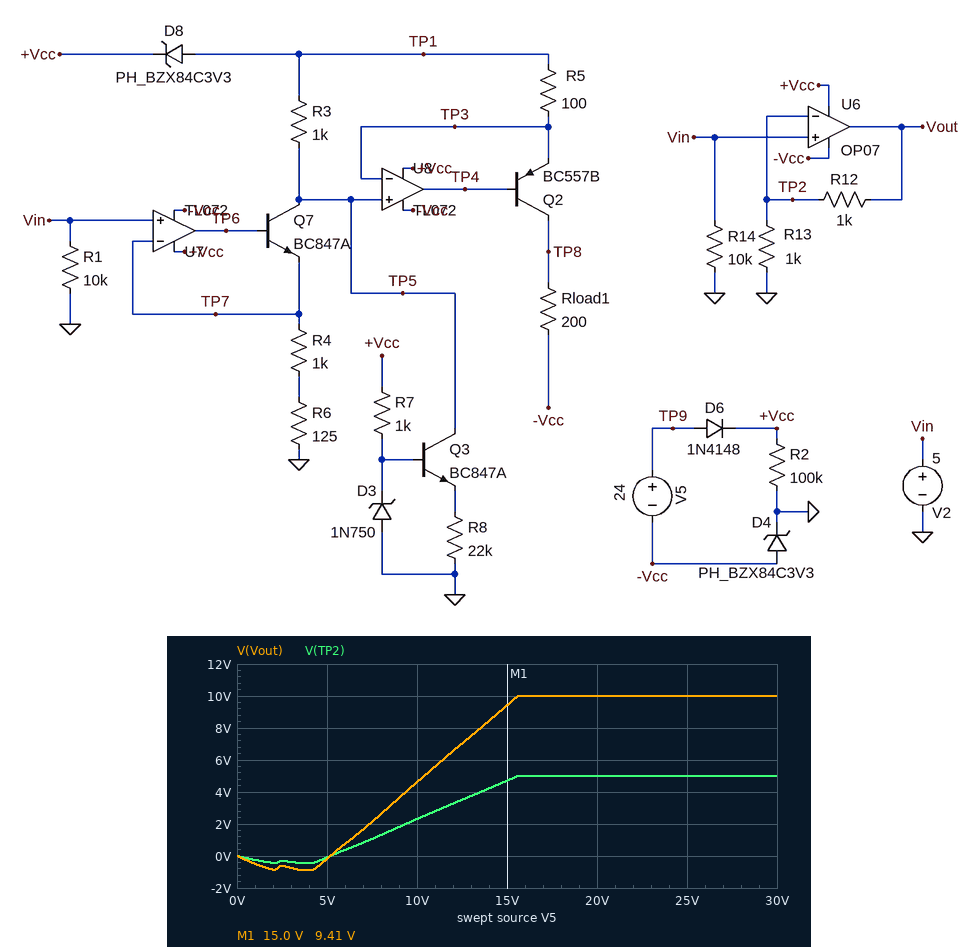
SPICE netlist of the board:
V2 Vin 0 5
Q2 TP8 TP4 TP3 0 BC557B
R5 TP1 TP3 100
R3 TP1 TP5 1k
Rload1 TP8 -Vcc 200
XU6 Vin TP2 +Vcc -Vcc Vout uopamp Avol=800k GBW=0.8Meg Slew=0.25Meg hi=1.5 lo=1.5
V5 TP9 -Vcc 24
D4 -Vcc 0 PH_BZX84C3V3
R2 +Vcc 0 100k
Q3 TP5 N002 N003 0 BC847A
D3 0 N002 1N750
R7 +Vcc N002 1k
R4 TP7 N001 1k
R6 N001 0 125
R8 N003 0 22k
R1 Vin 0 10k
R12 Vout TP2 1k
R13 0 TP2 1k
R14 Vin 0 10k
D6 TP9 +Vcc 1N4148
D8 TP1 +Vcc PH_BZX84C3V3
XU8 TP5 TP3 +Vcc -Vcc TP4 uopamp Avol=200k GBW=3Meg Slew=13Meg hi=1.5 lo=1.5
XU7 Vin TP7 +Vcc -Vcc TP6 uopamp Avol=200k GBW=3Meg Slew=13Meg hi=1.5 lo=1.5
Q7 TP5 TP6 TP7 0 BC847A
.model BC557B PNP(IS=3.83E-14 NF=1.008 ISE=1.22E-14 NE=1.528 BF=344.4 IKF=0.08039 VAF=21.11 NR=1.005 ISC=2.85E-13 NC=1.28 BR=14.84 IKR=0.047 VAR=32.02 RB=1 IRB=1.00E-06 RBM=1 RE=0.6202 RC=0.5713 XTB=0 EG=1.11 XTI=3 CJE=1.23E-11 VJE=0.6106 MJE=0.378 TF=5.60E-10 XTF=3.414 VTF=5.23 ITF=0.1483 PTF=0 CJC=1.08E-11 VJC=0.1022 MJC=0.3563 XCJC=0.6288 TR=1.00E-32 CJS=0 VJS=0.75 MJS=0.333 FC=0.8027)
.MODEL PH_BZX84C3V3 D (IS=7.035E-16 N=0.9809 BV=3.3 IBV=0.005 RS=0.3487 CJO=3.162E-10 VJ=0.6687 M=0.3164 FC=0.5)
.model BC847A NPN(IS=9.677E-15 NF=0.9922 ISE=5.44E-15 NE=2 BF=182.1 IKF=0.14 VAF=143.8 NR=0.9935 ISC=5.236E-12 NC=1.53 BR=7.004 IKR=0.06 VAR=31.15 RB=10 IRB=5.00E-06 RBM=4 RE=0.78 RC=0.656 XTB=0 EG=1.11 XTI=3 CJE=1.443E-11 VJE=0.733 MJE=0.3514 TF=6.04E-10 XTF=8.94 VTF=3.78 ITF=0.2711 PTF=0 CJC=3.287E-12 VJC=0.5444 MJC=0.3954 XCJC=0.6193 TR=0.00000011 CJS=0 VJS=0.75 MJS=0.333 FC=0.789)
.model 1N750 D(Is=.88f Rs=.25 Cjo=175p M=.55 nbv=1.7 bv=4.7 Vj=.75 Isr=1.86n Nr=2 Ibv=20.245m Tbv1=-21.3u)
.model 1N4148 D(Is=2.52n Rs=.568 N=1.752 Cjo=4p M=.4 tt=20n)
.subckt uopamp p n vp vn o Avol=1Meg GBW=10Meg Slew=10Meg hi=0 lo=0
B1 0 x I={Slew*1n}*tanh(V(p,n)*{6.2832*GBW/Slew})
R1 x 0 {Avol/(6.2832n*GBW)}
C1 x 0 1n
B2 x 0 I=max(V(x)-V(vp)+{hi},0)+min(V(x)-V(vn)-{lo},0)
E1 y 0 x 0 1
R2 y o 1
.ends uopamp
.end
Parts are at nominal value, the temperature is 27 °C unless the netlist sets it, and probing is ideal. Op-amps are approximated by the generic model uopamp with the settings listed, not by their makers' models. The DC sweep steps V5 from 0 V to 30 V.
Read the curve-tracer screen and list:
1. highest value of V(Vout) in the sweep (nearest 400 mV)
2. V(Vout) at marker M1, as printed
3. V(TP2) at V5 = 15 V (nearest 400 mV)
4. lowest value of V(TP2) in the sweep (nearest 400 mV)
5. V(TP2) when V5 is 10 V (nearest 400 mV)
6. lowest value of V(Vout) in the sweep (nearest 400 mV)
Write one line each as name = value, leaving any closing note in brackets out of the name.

highest value of V(Vout) in the sweep = 10.0 V
V(Vout) at marker M1, as printed = 9.41 V
V(TP2) at V5 = 15 V = 4.8 V
lowest value of V(TP2) in the sweep = -400 mV
V(TP2) when V5 is 10 V = 2.4 V
lowest value of V(Vout) in the sweep = -800 mV
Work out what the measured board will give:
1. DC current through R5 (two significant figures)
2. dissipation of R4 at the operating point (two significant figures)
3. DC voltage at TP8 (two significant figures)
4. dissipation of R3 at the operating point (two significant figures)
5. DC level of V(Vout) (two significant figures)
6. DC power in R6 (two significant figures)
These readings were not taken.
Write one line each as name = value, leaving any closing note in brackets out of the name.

DC current through R5 = 46 mA
dissipation of R4 at the operating point = 20 mW
DC voltage at TP8 = 5.8 V
dissipation of R3 at the operating point = 21 mW
DC level of V(Vout) = 10 V
DC power in R6 = 2.5 mW
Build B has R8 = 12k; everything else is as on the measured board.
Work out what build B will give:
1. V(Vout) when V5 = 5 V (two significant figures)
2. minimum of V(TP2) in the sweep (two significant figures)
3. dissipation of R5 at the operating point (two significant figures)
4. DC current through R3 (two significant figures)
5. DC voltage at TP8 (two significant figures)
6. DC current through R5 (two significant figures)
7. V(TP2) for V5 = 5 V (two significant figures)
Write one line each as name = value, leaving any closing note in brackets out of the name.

V(Vout) when V5 = 5 V = -190 mV
minimum of V(TP2) in the sweep = -430 mV
dissipation of R5 at the operating point = 230 mW
DC current through R3 = 4.8 mA
DC voltage at TP8 = 6.1 V
DC current through R5 = 48 mA
V(TP2) for V5 = 5 V = -95 mV
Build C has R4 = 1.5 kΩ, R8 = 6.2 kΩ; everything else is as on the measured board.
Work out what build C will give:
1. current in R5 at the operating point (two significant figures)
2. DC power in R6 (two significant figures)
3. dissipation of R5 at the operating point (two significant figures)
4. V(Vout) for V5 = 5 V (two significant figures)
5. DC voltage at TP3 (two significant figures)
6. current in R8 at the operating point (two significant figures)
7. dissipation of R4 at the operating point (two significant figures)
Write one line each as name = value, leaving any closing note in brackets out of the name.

current in R5 at the operating point = 37 mA
DC power in R6 = 1.2 mW
dissipation of R5 at the operating point = 140 mW
V(Vout) for V5 = 5 V = -210 mV
DC voltage at TP3 = 13 V
current in R8 at the operating point = 650 µA
dissipation of R4 at the operating point = 14 mW
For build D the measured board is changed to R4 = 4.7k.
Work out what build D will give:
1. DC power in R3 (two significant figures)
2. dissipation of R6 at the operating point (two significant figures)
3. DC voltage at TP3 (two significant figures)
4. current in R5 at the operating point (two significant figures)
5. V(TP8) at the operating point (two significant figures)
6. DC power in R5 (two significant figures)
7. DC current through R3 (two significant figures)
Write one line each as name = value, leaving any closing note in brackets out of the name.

DC power in R3 = 1.5 mW
dissipation of R6 at the operating point = 130 µW
DC voltage at TP3 = 15 V
current in R5 at the operating point = 12 mA
V(TP8) at the operating point = -910 mV
DC power in R5 = 15 mW
DC current through R3 = 1.2 mA
